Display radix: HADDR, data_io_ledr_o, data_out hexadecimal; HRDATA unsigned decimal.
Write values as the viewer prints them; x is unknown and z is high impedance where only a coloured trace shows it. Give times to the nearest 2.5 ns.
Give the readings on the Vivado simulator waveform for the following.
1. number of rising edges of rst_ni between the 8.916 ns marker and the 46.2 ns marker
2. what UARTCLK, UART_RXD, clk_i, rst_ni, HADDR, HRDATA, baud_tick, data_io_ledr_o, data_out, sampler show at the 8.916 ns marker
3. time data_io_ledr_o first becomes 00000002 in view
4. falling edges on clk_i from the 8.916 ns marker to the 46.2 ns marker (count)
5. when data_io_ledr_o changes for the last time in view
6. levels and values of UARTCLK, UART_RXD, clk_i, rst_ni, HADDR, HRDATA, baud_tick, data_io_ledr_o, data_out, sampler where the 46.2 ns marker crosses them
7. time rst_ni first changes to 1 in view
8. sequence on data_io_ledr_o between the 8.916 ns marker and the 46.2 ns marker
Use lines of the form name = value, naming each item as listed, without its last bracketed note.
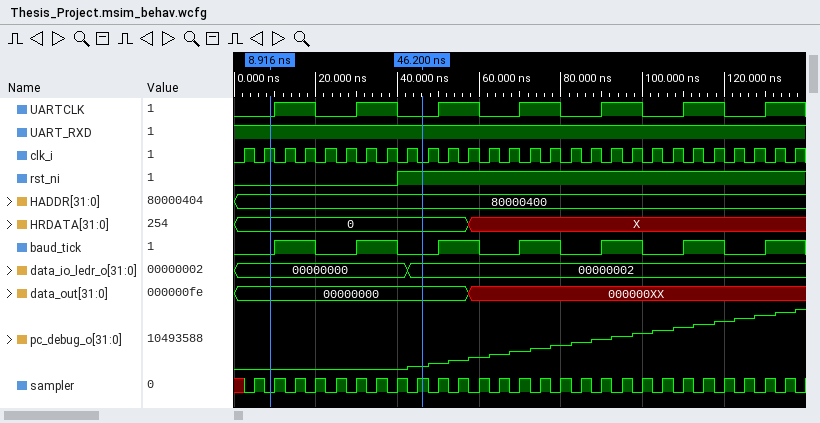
number of rising edges of rst_ni between the 8.916 ns marker and the 46.2 ns marker = 1
what UARTCLK, UART_RXD, clk_i, rst_ni, HADDR, HRDATA, baud_tick, data_io_ledr_o, data_out, sampler show at the 8.916 ns marker = UARTCLK=0, UART_RXD=1, clk_i=1, rst_ni=0, HADDR=80000400, HRDATA=0, baud_tick=0, data_io_ledr_o=00000000, data_out=00000000, sampler=0
time data_io_ledr_o first becomes 00000002 in view = 42.5 ns
falling edges on clk_i from the 8.916 ns marker to the 46.2 ns marker = 8
when data_io_ledr_o changes for the last time in view = 42.5 ns
levels and values of UARTCLK, UART_RXD, clk_i, rst_ni, HADDR, HRDATA, baud_tick, data_io_ledr_o, data_out, sampler where the 46.2 ns marker crosses them = UARTCLK=0, UART_RXD=1, clk_i=0, rst_ni=1, HADDR=80000400, HRDATA=0, baud_tick=0, data_io_ledr_o=00000002, data_out=00000000, sampler=1
time rst_ni first changes to 1 in view = 40 ns
sequence on data_io_ledr_o between the 8.916 ns marker and the 46.2 ns marker = 00000000, 00000002
